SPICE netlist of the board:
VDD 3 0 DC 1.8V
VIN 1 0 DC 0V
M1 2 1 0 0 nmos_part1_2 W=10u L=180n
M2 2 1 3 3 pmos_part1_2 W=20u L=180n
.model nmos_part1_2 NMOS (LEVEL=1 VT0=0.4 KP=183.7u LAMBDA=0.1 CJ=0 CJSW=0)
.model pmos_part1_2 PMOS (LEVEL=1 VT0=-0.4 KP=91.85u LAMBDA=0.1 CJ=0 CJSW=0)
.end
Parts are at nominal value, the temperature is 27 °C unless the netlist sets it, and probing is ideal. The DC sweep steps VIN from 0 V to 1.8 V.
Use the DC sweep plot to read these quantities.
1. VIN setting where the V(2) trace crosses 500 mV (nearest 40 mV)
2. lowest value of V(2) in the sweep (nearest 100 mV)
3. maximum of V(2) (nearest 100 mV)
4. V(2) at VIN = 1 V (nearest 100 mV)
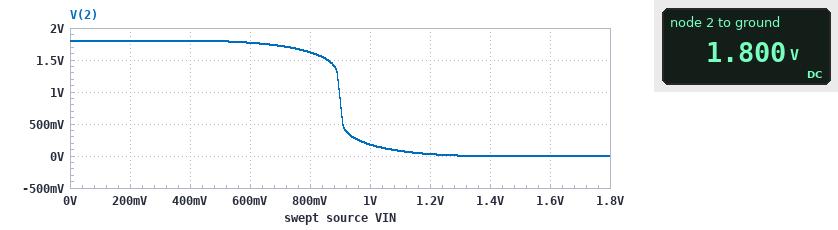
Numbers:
920 mV
0 V
1.8 V
200 mV
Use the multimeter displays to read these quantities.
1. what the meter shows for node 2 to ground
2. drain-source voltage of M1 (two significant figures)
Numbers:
1.800 V
1.8 V
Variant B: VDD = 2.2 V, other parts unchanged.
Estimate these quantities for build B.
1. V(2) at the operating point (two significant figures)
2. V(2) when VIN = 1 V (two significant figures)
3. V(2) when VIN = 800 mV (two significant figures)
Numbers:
2.2 V
1.9 V
2.1 V
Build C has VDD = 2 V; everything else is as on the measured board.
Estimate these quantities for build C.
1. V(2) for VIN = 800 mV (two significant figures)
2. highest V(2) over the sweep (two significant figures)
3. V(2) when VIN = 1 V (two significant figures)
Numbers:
1.9 V
2.0 V
1.0 V
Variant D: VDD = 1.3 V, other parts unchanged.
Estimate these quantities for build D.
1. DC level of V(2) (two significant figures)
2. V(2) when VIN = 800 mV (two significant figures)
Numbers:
1.3 V
14 mV
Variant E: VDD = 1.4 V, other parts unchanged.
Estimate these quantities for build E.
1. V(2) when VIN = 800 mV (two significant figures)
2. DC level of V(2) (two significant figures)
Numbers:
61 mV
1.4 V
